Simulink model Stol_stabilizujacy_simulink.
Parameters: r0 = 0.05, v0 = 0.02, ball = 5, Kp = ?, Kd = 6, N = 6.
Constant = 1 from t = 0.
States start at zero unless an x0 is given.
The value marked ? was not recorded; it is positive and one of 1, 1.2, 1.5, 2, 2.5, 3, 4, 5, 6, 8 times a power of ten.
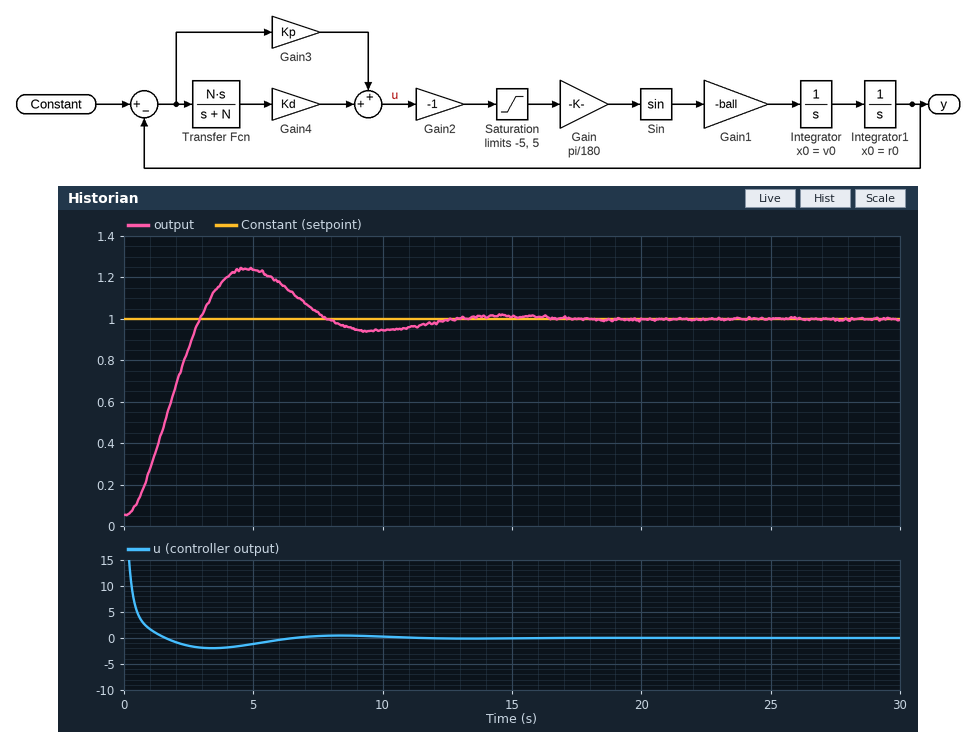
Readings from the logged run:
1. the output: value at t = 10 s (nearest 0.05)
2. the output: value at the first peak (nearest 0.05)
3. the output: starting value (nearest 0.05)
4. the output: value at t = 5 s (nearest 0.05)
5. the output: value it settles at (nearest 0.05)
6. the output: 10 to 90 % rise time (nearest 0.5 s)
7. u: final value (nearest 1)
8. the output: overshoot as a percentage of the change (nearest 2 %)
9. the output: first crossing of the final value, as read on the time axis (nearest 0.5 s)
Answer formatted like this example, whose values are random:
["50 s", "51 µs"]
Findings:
["0.95", "1.25", "0.05", "1.25", "1.00", "2.0 s", "0", "26 %", "3.0 s"]
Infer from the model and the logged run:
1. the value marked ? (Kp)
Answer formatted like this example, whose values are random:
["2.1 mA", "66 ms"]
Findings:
["5"]
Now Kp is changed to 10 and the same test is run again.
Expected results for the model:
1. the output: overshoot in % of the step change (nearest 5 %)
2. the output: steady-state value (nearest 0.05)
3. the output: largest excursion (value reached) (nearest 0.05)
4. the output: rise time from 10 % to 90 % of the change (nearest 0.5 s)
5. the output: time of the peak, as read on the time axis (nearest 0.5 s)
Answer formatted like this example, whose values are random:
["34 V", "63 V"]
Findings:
["35 %", "1.00", "1.35", "1.5 s", "3.5 s"]
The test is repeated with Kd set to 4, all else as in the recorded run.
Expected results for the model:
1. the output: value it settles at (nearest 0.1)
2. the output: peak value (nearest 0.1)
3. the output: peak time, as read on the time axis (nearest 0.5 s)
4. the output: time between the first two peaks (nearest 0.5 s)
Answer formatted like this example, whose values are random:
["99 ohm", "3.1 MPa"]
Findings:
["1.0", "1.4", "4.5 s", "9.5 s"]
